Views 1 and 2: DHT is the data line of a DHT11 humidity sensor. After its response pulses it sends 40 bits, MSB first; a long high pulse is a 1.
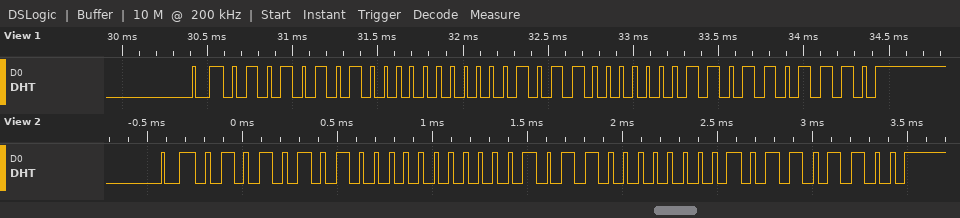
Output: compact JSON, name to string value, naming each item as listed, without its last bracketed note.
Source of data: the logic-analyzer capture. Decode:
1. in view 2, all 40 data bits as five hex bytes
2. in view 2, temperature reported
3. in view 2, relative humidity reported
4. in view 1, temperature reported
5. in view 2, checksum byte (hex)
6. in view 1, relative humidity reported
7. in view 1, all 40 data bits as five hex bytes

{"in view 2, all 40 data bits as five hex bytes": "55 00 16 01 6C", "in view 2, temperature reported": "22.1 °C", "in view 2, relative humidity reported": "85 %", "in view 1, temperature reported": "22.3 °C", "in view 2, checksum byte": "0x6C", "in view 1, relative humidity reported": "85 %", "in view 1, all 40 data bits as five hex bytes": "55 00 16 03 6E"}
